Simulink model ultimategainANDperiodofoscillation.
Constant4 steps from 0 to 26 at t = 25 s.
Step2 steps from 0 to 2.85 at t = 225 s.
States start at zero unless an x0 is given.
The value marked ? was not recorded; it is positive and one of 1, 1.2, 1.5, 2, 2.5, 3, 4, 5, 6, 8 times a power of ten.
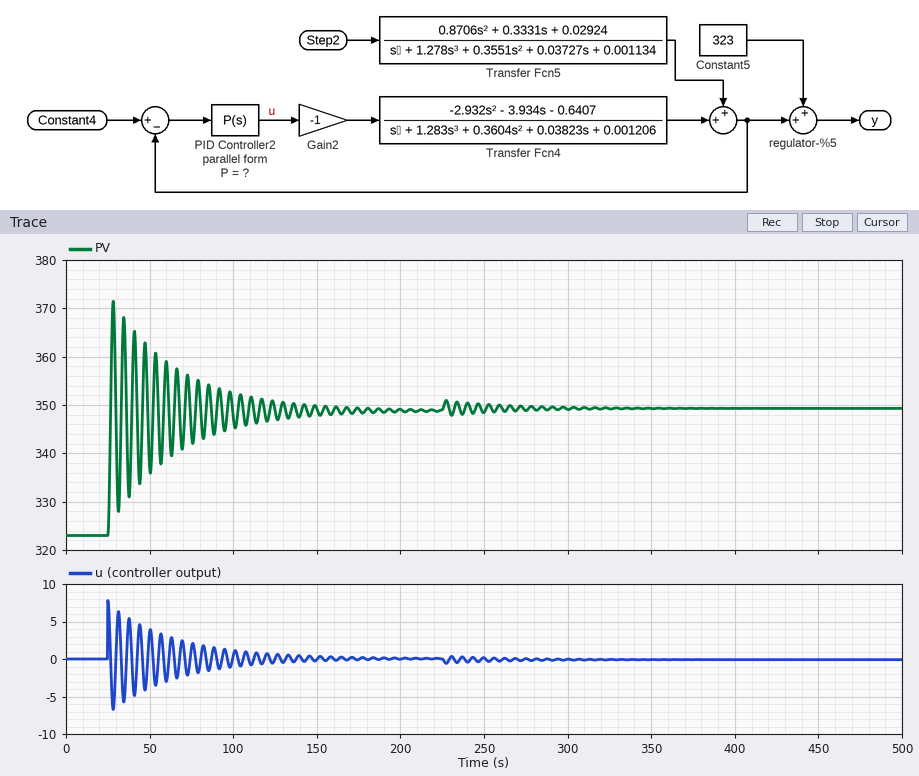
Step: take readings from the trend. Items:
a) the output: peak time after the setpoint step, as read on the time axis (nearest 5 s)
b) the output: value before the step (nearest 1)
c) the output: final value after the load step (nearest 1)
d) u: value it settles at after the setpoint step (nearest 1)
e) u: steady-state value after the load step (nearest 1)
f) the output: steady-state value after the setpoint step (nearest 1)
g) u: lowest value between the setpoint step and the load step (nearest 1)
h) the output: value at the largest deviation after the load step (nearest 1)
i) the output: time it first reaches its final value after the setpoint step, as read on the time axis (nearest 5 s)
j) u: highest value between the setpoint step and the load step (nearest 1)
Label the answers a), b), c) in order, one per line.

a) 30 s
b) 323
c) 349
d) 0
e) 0
f) 349
g) -7
h) 351
i) 25 s
j) 8
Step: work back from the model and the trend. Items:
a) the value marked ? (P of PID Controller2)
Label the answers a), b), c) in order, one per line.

a) 0.3
